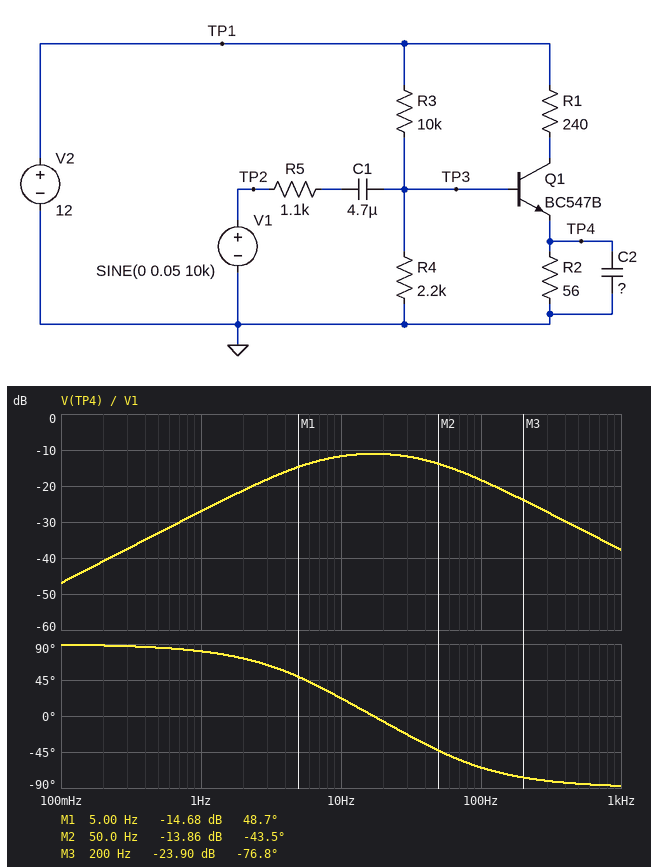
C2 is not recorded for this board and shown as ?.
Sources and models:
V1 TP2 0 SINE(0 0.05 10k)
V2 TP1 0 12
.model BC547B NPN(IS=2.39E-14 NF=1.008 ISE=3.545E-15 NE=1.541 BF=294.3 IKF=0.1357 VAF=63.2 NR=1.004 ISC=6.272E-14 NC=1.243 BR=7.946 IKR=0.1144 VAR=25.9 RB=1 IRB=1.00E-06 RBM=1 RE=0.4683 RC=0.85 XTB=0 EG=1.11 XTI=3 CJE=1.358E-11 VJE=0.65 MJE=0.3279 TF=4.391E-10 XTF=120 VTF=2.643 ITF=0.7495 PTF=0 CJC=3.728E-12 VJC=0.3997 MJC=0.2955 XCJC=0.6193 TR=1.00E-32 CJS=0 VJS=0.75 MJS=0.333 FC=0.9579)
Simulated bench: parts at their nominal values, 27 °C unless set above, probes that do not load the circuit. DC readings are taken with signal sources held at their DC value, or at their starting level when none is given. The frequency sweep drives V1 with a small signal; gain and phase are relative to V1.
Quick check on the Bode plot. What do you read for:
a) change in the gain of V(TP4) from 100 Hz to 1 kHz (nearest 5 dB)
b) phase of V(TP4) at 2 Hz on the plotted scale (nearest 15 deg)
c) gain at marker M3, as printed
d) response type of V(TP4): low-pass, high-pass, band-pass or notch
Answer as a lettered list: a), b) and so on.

a) -20 dB
b) 75 deg
c) -23.90 dB
d) band-pass
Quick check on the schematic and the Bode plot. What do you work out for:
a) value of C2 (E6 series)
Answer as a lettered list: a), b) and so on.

a) 1.5 mF
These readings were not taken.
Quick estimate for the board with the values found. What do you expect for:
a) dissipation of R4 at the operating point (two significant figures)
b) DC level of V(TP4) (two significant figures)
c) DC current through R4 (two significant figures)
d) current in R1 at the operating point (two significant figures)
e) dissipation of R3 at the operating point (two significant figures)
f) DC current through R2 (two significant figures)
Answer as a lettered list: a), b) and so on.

a) 1.8 mW
b) 1.3 V
c) 910 µA
d) 23 mA
e) 10 mW
f) 23 mA
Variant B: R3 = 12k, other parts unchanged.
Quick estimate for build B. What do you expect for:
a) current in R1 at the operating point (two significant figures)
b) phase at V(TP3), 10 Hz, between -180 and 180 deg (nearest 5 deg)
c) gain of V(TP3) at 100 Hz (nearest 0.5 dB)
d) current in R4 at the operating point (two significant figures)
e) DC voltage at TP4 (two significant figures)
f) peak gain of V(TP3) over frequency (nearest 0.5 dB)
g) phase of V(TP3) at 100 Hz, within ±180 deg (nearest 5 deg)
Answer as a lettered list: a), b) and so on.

a) 18 mA
b) 35 deg
c) -11.0 dB
d) 790 µA
e) 1.0 V
f) -10.0 dB
g) 0 deg
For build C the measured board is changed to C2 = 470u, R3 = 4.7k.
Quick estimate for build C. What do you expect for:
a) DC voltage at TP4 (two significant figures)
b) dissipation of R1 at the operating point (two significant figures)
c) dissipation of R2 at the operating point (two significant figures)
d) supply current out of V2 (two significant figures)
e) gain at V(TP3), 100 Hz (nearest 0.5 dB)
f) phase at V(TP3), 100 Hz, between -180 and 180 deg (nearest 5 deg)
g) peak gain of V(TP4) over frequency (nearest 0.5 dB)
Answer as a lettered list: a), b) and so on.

a) 2.3 V
b) 380 mW
c) 92 mW
d) 42 mA
e) -42.5 dB
f) -15 deg
g) -40.0 dB
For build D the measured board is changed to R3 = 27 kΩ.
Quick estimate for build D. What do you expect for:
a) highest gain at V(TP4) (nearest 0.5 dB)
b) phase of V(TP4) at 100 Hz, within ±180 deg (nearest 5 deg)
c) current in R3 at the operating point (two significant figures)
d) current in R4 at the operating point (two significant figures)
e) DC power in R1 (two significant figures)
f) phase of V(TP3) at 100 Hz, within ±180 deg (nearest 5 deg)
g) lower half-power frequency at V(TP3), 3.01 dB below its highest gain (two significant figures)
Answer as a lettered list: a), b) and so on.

a) -12.0 dB
b) -75 deg
c) 410 µA
d) 400 µA
e) 3.3 mW
f) 5 deg
g) 12 Hz
